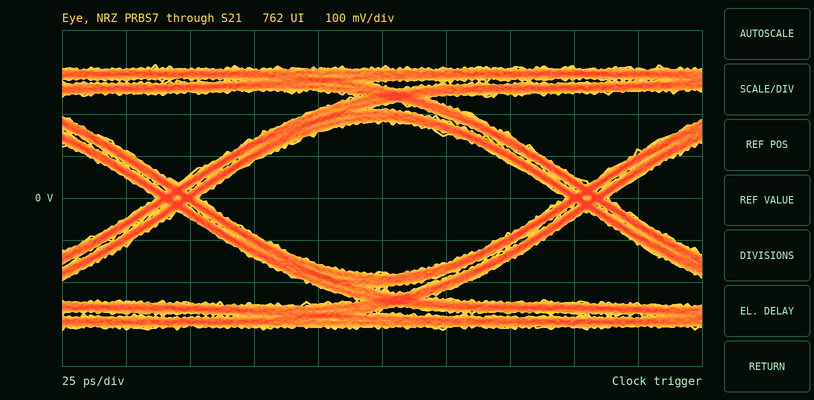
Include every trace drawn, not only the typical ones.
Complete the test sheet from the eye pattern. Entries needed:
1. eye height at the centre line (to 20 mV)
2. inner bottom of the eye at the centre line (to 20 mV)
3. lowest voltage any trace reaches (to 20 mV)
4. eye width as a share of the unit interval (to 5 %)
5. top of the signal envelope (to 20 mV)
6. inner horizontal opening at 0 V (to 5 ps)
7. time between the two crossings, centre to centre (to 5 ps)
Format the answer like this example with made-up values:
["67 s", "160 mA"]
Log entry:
["360 mV", "-180 mV", "-320 mV", "90 %", "320 mV", "145 ps", "160 ps"]
